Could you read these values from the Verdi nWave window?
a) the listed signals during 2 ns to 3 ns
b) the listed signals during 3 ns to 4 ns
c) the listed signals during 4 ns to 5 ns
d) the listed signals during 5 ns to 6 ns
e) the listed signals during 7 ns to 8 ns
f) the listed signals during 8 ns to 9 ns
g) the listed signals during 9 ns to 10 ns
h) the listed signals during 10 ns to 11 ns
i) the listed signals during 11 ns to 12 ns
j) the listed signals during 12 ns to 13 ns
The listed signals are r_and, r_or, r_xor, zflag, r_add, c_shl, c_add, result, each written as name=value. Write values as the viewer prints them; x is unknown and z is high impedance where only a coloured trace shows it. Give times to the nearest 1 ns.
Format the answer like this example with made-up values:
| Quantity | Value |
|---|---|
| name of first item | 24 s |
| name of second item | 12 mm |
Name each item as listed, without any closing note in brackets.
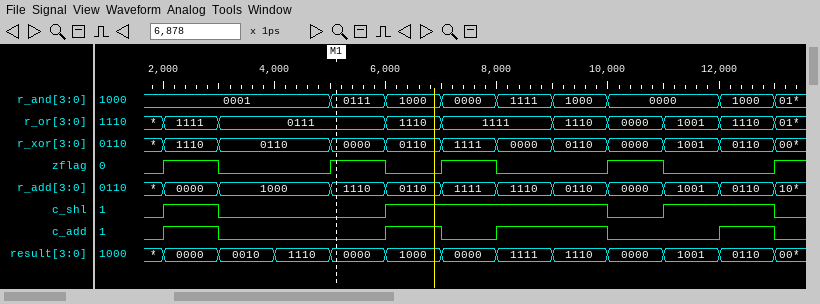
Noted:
| Quantity | Value |
|---|---|
| the listed signals during 2 ns to 3 ns | r_and=0001, r_or=1111, r_xor=1110, zflag=1, r_add=0000, c_shl=1, c_add=1, result=0000 |
| the listed signals during 3 ns to 4 ns | r_and=0001, r_or=0111, r_xor=0110, zflag=0, r_add=1000, c_shl=0, c_add=0, result=0010 |
| the listed signals during 4 ns to 5 ns | r_and=0001, r_or=0111, r_xor=0110, zflag=0, r_add=1000, c_shl=0, c_add=0, result=1110 |
| the listed signals during 5 ns to 6 ns | r_and=0111, r_or=0111, r_xor=0000, zflag=1, r_add=1110, c_shl=0, c_add=0, result=0000 |
| the listed signals during 7 ns to 8 ns | r_and=0000, r_or=1111, r_xor=1111, zflag=1, r_add=1111, c_shl=1, c_add=0, result=0000 |
| the listed signals during 8 ns to 9 ns | r_and=1111, r_or=1111, r_xor=0000, zflag=0, r_add=1110, c_shl=1, c_add=1, result=1111 |
| the listed signals during 9 ns to 10 ns | r_and=1000, r_or=1110, r_xor=0110, zflag=0, r_add=0110, c_shl=1, c_add=1, result=1110 |
| the listed signals during 10 ns to 11 ns | r_and=0000, r_or=0000, r_xor=0000, zflag=1, r_add=0000, c_shl=0, c_add=0, result=0000 |
| the listed signals during 11 ns to 12 ns | r_and=0000, r_or=1001, r_xor=1001, zflag=0, r_add=1001, c_shl=1, c_add=0, result=1001 |
| the listed signals during 12 ns to 13 ns | r_and=1000, r_or=1110, r_xor=0110, zflag=0, r_add=0110, c_shl=1, c_add=1, result=0110 |
